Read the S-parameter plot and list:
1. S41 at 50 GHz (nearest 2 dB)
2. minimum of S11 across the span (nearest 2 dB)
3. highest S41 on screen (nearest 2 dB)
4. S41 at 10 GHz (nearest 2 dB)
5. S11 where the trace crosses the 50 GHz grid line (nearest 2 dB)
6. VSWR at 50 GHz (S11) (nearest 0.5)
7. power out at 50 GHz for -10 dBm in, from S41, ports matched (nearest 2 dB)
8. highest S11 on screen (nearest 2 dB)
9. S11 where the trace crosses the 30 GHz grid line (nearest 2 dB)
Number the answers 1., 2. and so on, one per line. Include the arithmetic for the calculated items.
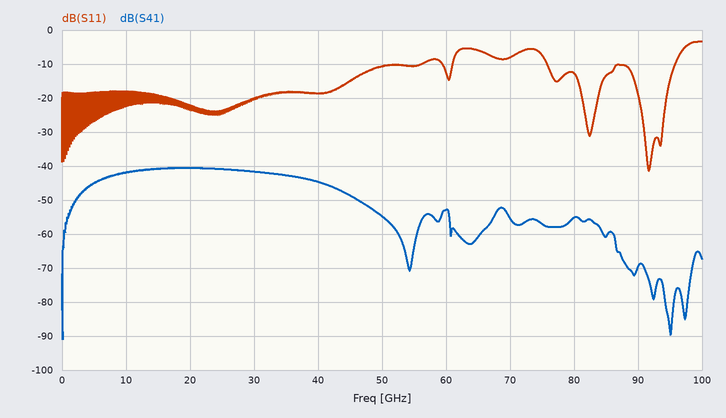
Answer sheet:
1. -54 dB
2. -42 dB
3. -40 dB
4. -42 dB
5. -10 dB
6. |Γ| = 10^(-10/20) = 0.3162; VSWR = (1 + 0.3162)/(1 − 0.3162) ≈ 1.92, so 2.0 to the nearest 0.5
7. -10 dBm + (-54 dB) = -64 dBm
8. -4 dB
9. -20 dB
